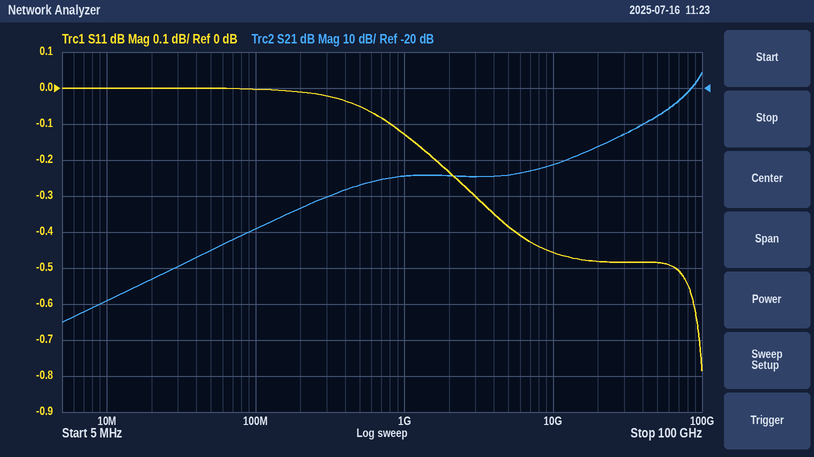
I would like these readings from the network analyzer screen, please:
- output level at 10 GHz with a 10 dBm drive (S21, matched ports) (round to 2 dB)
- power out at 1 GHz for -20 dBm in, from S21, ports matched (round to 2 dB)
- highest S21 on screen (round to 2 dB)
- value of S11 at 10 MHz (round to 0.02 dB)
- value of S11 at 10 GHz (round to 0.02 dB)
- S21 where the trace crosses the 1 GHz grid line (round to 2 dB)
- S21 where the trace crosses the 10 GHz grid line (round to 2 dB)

-32 dBm
-64 dBm
-16 dB
0.00 dB
-0.46 dB
-44 dB
-42 dB
